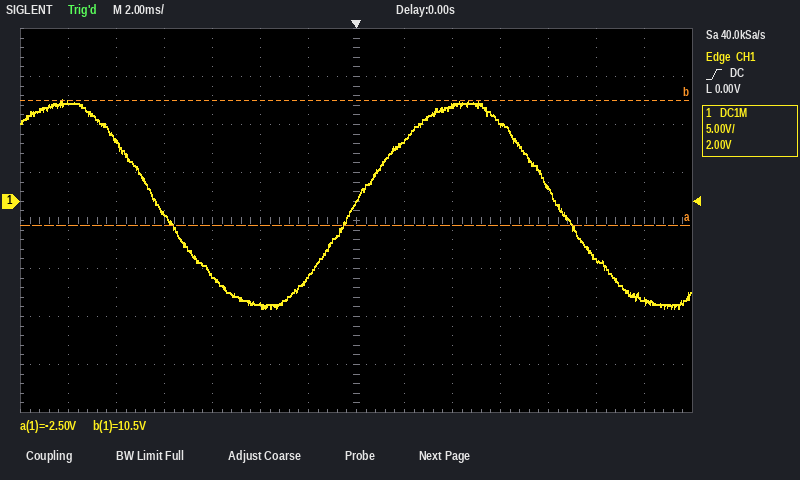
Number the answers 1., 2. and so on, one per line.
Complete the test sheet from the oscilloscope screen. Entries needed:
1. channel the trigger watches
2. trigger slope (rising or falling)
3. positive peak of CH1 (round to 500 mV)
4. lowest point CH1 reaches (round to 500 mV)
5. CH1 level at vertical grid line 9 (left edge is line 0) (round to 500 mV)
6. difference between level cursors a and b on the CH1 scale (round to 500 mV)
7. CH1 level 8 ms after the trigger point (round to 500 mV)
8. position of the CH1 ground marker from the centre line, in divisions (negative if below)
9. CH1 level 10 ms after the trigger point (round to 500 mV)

1. CH1
2. rising
3. 10.5 V
4. -11.0 V
5. 10.0 V
6. 13.0 V
7. 1.5 V
8. +0.4 div
9. -6.0 V
